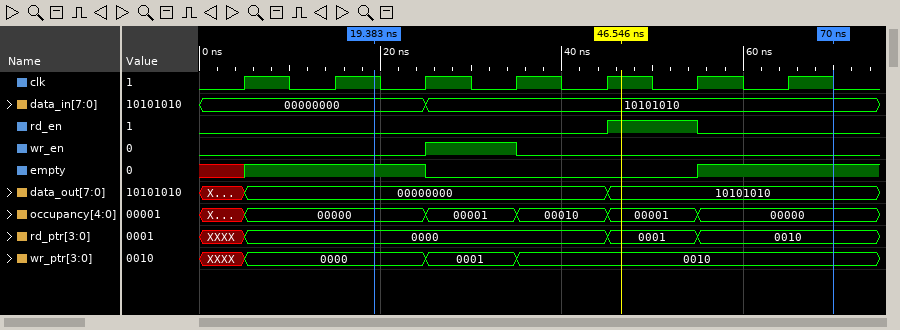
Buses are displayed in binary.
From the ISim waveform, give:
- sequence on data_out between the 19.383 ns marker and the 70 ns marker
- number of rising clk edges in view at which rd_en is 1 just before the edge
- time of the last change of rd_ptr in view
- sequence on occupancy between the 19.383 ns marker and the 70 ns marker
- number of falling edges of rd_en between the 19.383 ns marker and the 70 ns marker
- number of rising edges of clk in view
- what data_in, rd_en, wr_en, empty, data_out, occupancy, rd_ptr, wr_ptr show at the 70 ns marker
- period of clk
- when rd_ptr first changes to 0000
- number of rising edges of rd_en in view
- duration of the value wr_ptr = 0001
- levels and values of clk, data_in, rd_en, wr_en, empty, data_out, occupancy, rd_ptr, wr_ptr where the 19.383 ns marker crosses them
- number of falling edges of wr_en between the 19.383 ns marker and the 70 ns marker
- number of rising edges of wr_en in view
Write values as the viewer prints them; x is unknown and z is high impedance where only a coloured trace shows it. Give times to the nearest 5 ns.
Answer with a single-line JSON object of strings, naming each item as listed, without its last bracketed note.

{"sequence on data_out between the 19.383 ns marker and the 70 ns marker": "00000000, 10101010", "number of rising clk edges in view at which rd_en is 1 just before the edge": "1", "time of the last change of rd_ptr in view": "55 ns", "sequence on occupancy between the 19.383 ns marker and the 70 ns marker": "00000, 00001, 00010, 00001, 00000", "number of falling edges of rd_en between the 19.383 ns marker and the 70 ns marker": "1", "number of rising edges of clk in view": "7", "what data_in, rd_en, wr_en, empty, data_out, occupancy, rd_ptr, wr_ptr show at the 70 ns marker": "data_in=10101010, rd_en=0, wr_en=0, empty=1, data_out=10101010, occupancy=00000, rd_ptr=0010, wr_ptr=0010", "period of clk": "10 ns", "when rd_ptr first changes to 0000": "5 ns", "number of rising edges of rd_en in view": "1", "duration of the value wr_ptr = 0001": "10 ns", "levels and values of clk, data_in, rd_en, wr_en, empty, data_out, occupancy, rd_ptr, wr_ptr where the 19.383 ns marker crosses them": "clk=1, data_in=00000000, rd_en=0, wr_en=0, empty=1, data_out=00000000, occupancy=00000, rd_ptr=0000, wr_ptr=0000", "number of falling edges of wr_en between the 19.383 ns marker and the 70 ns marker": "1", "number of rising edges of wr_en in view": "1"}
